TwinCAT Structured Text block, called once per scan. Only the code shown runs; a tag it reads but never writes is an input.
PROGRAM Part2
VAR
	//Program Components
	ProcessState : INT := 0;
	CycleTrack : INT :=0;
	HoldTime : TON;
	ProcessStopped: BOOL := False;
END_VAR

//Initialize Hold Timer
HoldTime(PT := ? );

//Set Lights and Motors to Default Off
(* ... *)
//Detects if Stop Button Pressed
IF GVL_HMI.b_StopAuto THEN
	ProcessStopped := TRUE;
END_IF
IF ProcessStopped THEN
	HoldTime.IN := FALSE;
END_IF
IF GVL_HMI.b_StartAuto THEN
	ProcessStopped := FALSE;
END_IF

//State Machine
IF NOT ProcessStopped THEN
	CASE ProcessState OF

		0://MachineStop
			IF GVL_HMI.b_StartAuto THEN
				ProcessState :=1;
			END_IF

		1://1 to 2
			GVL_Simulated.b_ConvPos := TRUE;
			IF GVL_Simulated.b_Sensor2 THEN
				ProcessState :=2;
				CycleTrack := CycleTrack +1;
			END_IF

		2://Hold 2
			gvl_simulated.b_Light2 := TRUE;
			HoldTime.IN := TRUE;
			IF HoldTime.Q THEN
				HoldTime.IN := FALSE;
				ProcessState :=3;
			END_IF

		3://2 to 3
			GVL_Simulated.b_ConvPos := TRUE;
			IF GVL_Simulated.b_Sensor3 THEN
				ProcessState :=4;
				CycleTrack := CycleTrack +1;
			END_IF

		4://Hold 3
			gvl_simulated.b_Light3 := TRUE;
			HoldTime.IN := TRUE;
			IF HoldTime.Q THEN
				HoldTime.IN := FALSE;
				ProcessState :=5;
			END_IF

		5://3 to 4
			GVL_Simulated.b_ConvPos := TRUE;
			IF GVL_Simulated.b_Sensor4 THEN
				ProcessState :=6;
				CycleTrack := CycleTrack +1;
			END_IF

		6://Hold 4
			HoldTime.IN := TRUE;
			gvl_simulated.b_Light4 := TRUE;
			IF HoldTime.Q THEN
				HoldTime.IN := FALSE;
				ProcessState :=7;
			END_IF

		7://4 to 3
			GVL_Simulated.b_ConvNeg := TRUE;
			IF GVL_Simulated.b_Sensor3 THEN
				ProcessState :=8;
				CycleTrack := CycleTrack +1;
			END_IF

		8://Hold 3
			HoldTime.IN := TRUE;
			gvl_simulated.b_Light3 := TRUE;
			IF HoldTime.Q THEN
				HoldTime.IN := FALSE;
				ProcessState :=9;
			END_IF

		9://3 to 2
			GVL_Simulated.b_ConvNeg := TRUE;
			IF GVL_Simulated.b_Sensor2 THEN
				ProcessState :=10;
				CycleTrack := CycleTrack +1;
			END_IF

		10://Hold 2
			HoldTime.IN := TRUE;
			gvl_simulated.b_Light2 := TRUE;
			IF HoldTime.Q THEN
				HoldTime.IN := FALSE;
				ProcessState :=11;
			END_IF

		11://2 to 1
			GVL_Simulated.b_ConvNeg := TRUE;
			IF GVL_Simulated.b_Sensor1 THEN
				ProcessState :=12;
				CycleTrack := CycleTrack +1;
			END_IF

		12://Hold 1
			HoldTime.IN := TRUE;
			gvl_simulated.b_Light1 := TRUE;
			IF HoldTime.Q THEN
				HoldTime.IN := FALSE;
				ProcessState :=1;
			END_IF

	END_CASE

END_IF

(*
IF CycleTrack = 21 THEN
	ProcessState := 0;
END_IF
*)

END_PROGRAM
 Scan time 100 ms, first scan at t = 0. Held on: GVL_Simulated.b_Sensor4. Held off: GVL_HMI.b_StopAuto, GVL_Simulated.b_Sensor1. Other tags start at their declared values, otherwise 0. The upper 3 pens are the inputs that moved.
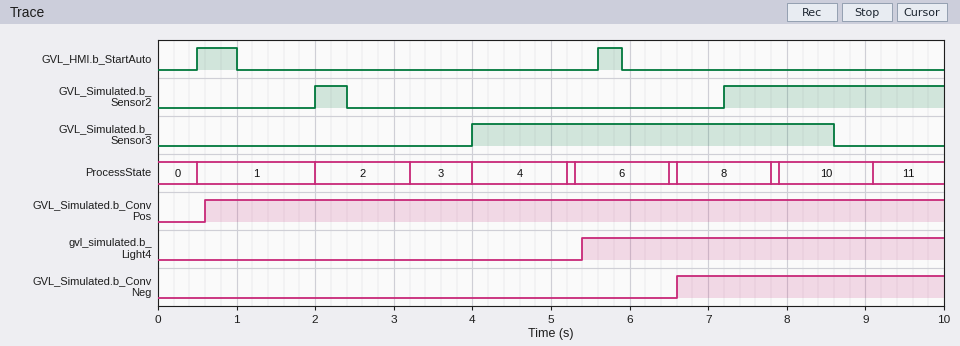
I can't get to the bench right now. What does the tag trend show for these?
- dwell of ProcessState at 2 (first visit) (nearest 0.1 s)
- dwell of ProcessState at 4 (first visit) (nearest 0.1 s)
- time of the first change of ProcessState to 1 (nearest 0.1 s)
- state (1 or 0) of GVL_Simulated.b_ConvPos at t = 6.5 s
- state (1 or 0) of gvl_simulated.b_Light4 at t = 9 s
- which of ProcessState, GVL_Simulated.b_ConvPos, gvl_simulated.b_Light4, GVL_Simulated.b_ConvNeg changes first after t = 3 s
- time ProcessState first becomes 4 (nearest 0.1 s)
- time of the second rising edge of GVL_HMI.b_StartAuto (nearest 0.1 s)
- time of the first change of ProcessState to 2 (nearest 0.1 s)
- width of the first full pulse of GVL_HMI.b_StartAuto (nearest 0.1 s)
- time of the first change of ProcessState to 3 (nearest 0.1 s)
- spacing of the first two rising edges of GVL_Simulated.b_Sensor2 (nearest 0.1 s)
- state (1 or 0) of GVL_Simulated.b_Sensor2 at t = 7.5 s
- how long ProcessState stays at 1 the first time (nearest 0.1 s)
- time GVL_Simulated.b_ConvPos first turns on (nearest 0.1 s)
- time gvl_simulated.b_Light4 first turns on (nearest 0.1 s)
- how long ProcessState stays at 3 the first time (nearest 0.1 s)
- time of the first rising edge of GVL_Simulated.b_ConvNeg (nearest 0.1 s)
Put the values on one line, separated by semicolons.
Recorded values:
1.2 s; 1.2 s; 0.5 s; 1; 1; ProcessState; 4.0 s; 5.6 s; 2.0 s; 0.5 s; 3.2 s; 5.2 s; 1; 1.5 s; 0.6 s; 5.4 s; 0.8 s; 6.6 s
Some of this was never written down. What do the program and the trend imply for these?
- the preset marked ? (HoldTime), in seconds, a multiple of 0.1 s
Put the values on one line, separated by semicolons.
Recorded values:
1.0 s
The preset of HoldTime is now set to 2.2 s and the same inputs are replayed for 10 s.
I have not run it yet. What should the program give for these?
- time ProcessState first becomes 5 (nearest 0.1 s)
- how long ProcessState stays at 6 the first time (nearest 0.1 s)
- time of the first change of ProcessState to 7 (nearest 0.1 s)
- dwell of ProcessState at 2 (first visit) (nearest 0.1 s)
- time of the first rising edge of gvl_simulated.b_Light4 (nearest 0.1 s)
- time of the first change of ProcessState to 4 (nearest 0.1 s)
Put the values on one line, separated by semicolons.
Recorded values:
6.9 s; 2.4 s; 9.4 s; 2.4 s; 7.1 s; 4.5 s
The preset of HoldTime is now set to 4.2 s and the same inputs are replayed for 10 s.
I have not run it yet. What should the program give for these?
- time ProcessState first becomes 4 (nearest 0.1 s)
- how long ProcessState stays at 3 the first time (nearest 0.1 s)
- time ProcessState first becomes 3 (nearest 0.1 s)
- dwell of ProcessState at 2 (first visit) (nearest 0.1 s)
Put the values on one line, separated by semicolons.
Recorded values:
6.5 s; 0.1 s; 6.4 s; 4.4 s
